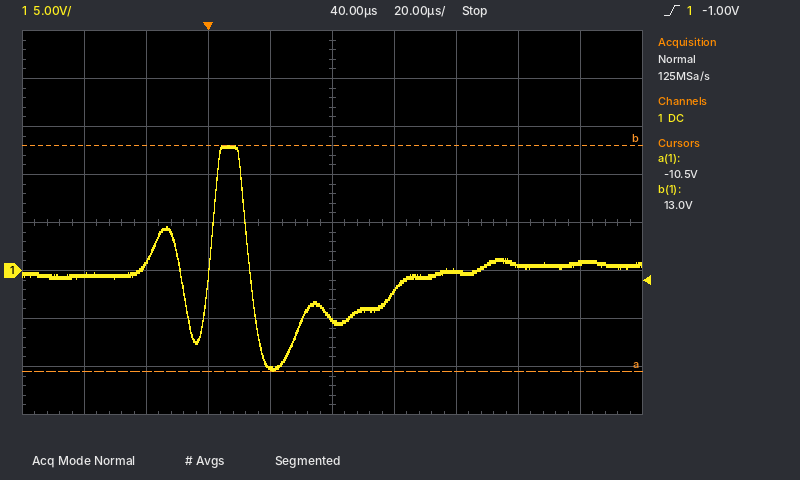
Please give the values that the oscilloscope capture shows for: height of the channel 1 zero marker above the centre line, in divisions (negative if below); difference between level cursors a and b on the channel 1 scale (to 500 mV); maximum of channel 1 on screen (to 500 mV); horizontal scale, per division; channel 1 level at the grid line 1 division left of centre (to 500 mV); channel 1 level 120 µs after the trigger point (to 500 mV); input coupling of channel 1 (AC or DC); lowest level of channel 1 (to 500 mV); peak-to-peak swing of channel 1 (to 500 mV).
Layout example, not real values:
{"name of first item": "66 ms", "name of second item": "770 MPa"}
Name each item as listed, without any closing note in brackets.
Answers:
{"height of the channel 1 zero marker above the centre line, in divisions": "-1.0 div", "difference between level cursors a and b on the channel 1 scale": "23.5 V", "maximum of channel 1 on screen": "13.0 V", "horizontal scale, per division": "20 µs", "channel 1 level at the grid line 1 division left of centre": "-10.0 V", "channel 1 level 120 µs after the trigger point": "1.0 V", "input coupling of channel 1": "DC", "lowest level of channel 1": "-10.5 V", "peak-to-peak swing of channel 1": "23.5 V"}
